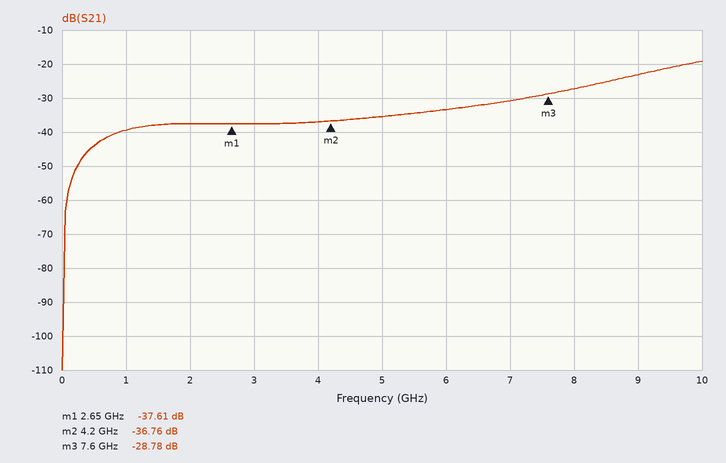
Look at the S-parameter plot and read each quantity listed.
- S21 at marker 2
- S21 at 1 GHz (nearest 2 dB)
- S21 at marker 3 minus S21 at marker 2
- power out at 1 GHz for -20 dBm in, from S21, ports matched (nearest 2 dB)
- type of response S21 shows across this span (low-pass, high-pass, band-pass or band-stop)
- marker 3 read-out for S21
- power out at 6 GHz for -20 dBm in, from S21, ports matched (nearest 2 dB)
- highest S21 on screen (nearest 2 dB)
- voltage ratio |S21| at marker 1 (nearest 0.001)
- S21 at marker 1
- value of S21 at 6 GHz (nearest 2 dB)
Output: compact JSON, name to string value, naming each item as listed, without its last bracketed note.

{"S21 at marker 2": "-36.76 dB", "S21 at 1 GHz": "-40 dB", "S21 at marker 3 minus S21 at marker 2": "7.98 dB", "power out at 1 GHz for -20 dBm in, from S21, ports matched": "-60 dBm", "type of response S21 shows across this span": "high-pass", "marker 3 read-out for S21": "-28.78 dB", "power out at 6 GHz for -20 dBm in, from S21, ports matched": "-54 dBm", "highest S21 on screen": "-20 dB", "voltage ratio |S21| at marker 1": "0.013", "S21 at marker 1": "-37.61 dB", "value of S21 at 6 GHz": "-34 dB"}
